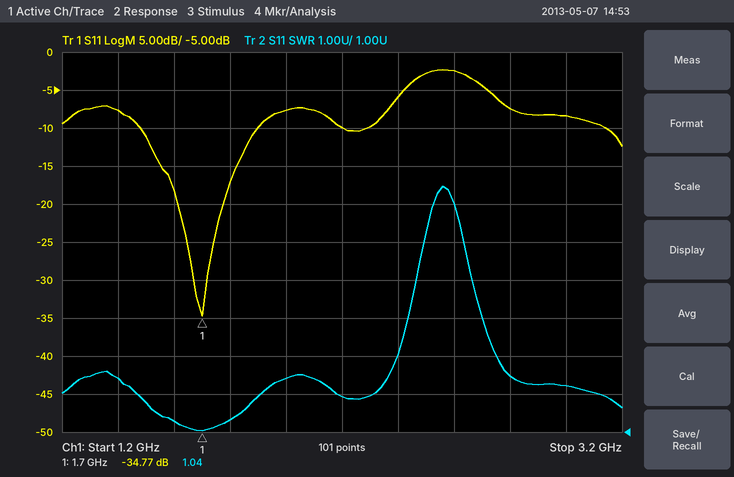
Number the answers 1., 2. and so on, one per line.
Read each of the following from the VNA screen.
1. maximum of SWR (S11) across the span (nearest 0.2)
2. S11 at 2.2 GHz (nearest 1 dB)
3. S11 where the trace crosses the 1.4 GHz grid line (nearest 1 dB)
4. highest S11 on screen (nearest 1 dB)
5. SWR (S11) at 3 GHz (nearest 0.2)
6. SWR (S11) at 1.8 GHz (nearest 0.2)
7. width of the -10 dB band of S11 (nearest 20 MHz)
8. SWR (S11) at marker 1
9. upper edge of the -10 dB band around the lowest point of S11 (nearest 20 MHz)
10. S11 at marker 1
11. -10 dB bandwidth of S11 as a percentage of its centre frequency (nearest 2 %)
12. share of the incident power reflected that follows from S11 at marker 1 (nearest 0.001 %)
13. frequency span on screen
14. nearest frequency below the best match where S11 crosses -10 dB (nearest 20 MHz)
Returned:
1. 7.4
2. -10 dB
3. -8 dB
4. -2 dB
5. 2.2
6. 1.4
7. 420 MHz
8. 1.04
9. 1.90 GHz
10. -34.77 dB
11. 24 %
12. 0.033 %
13. 2 GHz
14. 1.48 GHz
